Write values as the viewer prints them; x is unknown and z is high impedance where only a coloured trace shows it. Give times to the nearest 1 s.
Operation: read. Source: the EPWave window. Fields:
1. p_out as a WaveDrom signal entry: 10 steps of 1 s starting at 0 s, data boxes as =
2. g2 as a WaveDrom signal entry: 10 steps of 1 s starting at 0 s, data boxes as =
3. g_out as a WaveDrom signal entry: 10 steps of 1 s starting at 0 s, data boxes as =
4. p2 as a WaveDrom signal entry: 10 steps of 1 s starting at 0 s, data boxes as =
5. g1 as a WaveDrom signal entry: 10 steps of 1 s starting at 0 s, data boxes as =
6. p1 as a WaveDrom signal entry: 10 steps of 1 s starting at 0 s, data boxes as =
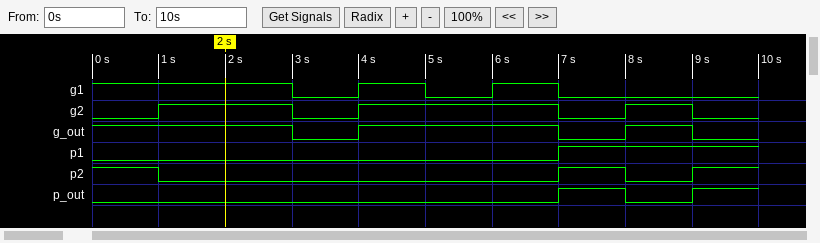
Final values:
{name: 'p_out', wave: '0......101'}
{name: 'g2', wave: '01.01..010'}
{name: 'g_out', wave: '1..01..010'}
{name: 'p2', wave: '10.....101'}
{name: 'g1', wave: '1..01010..'}
{name: 'p1', wave: '0......1..'}
